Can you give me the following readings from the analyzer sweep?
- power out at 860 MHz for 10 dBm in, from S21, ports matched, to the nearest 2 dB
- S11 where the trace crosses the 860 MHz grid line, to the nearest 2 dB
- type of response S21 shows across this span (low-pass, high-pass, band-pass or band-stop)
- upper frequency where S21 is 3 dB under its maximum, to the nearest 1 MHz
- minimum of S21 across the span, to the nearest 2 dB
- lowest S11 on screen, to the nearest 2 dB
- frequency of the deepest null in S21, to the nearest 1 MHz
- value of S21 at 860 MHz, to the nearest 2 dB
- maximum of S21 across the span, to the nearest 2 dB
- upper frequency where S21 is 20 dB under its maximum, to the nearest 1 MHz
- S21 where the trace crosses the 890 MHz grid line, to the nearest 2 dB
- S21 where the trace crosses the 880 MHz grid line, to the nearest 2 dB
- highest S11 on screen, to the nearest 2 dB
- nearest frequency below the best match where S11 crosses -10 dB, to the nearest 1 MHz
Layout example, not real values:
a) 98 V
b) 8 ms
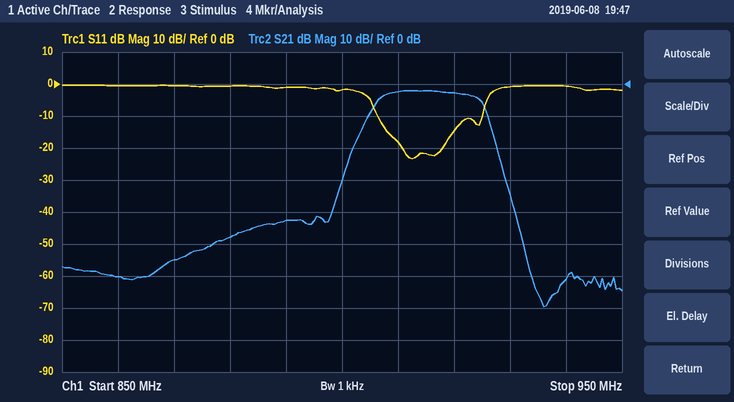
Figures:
a) -50 dBm
b) 0 dB
c) band-pass
d) 925 MHz
e) -70 dB
f) -24 dB
g) 936 MHz
h) -60 dB
i) -2 dB
j) 928 MHz
k) -42 dB
l) -48 dB
m) 0 dB
n) 906 MHz
